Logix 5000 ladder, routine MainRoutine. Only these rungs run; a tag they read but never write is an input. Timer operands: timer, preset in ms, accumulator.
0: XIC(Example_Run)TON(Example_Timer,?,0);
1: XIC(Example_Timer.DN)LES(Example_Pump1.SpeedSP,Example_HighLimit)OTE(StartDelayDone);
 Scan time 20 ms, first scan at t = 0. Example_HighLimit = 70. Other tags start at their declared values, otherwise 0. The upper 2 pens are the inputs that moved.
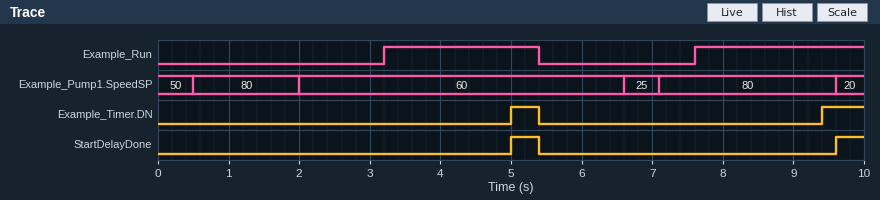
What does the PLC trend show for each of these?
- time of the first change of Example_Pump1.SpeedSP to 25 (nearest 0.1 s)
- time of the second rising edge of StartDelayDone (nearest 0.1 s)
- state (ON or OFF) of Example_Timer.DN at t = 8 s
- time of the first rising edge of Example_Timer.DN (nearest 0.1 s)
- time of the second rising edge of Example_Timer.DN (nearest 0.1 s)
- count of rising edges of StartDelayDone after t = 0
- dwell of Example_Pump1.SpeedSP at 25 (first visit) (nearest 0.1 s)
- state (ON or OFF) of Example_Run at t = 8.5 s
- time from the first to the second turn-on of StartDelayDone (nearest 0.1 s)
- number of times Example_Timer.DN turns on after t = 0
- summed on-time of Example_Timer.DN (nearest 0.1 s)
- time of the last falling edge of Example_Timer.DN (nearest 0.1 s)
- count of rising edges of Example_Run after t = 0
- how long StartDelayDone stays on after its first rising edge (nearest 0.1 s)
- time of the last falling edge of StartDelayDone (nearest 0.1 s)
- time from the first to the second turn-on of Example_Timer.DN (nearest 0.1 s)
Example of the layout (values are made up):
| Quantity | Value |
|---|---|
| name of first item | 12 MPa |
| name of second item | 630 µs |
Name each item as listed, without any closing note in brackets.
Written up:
| Quantity | Value |
|---|---|
| time of the first change of Example_Pump1.SpeedSP to 25 | 6.6 s |
| time of the second rising edge of StartDelayDone | 9.6 s |
| state (ON or OFF) of Example_Timer.DN at t = 8 s | OFF |
| time of the first rising edge of Example_Timer.DN | 5.0 s |
| time of the second rising edge of Example_Timer.DN | 9.4 s |
| count of rising edges of StartDelayDone after t = 0 | 2 |
| dwell of Example_Pump1.SpeedSP at 25 (first visit) | 0.5 s |
| state (ON or OFF) of Example_Run at t = 8.5 s | ON |
| time from the first to the second turn-on of StartDelayDone | 4.6 s |
| number of times Example_Timer.DN turns on after t = 0 | 2 |
| summed on-time of Example_Timer.DN | 1.0 s |
| time of the last falling edge of Example_Timer.DN | 5.4 s |
| count of rising edges of Example_Run after t = 0 | 2 |
| how long StartDelayDone stays on after its first rising edge | 0.4 s |
| time of the last falling edge of StartDelayDone | 5.4 s |
| time from the first to the second turn-on of Example_Timer.DN | 4.4 s |
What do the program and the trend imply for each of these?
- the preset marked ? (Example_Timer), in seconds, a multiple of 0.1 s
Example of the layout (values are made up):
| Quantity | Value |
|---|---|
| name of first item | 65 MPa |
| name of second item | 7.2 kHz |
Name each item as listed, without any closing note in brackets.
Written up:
| Quantity | Value |
|---|---|
| the preset marked ? (Example_Timer), in seconds, a multiple of 0.1 s | 1.8 s |
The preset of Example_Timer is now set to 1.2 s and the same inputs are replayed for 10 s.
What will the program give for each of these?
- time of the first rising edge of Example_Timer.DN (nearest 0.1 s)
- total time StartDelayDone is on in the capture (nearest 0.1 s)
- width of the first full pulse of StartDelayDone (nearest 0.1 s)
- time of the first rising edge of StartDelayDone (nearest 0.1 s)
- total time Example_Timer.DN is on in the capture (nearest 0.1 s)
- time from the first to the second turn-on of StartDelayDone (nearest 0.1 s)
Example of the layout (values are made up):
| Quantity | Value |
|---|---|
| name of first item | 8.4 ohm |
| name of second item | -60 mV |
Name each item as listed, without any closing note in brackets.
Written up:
| Quantity | Value |
|---|---|
| time of the first rising edge of Example_Timer.DN | 4.4 s |
| total time StartDelayDone is on in the capture | 1.4 s |
| width of the first full pulse of StartDelayDone | 1.0 s |
| time of the first rising edge of StartDelayDone | 4.4 s |
| total time Example_Timer.DN is on in the capture | 2.2 s |
| time from the first to the second turn-on of StartDelayDone | 5.2 s |
